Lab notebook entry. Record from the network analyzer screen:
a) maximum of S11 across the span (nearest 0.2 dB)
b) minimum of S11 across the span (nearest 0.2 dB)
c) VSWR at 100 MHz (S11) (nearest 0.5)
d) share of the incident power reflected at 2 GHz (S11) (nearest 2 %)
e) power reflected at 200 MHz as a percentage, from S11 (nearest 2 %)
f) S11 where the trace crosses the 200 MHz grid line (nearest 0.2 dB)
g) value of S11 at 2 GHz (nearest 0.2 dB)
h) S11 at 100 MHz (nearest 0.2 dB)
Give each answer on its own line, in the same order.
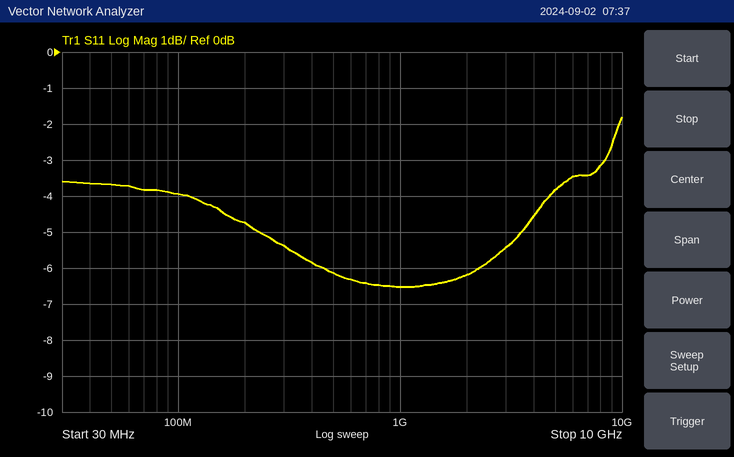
-1.8 dB
-6.6 dB
4.5
24 %
34 %
-4.8 dB
-6.2 dB
-4.0 dB
